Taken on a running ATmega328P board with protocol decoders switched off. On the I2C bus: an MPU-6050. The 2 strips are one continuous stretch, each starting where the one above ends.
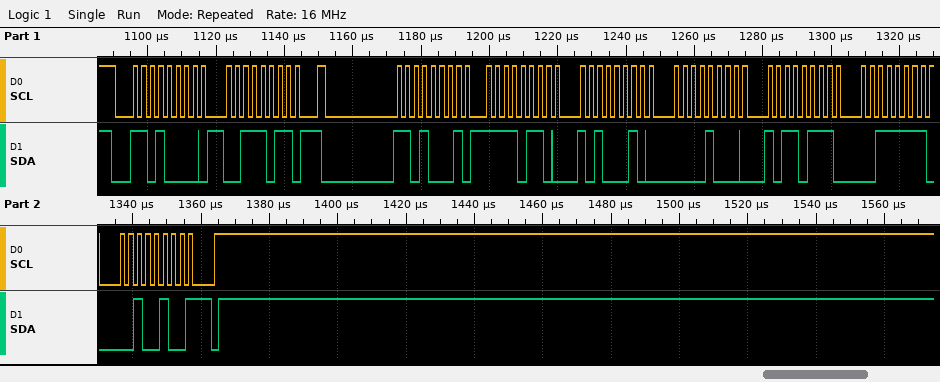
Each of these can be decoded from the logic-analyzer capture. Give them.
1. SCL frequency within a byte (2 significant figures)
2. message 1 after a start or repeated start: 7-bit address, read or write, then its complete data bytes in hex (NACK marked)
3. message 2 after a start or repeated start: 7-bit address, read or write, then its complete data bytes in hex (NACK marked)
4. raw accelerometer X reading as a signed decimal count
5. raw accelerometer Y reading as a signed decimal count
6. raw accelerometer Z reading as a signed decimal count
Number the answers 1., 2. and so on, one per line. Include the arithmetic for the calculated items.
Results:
1. 400 kHz
2. 0x68 write: 3B
3. 0x68 read: F6 A2 08 B7 3F 24 NACK
4. 0xF6A2 = -2398
5. 0x08B7 = 2231
6. 0x3F24 = 16164
